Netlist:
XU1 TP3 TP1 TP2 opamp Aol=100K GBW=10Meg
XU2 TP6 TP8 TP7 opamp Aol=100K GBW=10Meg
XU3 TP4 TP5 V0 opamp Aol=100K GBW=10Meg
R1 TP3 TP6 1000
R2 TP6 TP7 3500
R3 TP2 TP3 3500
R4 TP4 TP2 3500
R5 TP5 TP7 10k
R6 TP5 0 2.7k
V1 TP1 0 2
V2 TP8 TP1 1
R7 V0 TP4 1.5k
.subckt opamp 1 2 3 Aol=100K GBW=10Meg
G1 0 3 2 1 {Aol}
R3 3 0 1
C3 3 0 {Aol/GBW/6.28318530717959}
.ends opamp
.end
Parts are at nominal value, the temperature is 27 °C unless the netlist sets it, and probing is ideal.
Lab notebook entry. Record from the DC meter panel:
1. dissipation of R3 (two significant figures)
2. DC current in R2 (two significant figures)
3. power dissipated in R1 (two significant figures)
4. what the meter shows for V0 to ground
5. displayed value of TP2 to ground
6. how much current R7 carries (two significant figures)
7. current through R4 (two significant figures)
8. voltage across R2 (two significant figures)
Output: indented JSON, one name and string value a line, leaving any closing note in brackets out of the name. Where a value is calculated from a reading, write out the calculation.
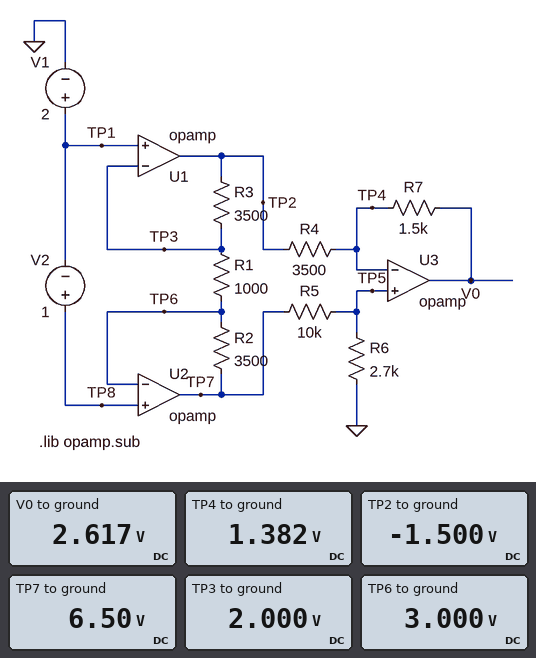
{
  "dissipation of R3": "(2 V - (-1.5 V))^2 / 3.5 kΩ = 3.5 mW",
  "DC current in R2": "(6.5 V - 3 V) / 3.5 kΩ = 1.0 mA",
  "power dissipated in R1": "(3 V - 2 V)^2 / 1 kΩ = 1.0 mW",
  "what the meter shows for V0 to ground": "2.617 V",
  "displayed value of TP2 to ground": "-1.500 V",
  "how much current R7 carries": "(2.617 V - 1.382 V) / 1.5 kΩ = 820 µA",
  "current through R4": "(1.382 V - (-1.5 V)) / 3.5 kΩ = 820 µA",
  "voltage across R2": "6.5 V - 3 V = 3.5 V"
}
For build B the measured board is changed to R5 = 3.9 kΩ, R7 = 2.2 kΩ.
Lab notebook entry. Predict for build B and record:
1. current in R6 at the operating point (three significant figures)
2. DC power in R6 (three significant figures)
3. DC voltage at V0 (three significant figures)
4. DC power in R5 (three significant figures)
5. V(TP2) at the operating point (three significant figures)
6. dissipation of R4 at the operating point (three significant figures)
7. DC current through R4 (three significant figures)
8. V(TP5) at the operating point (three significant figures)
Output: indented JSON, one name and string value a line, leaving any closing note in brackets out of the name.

{
  "current in R6 at the operating point": "985 µA",
  "DC power in R6": "2.62 mW",
  "DC voltage at V0": "5.27 V",
  "DC power in R5": "3.78 mW",
  "V(TP2) at the operating point": "-1.50 V",
  "dissipation of R4 at the operating point": "4.94 mW",
  "DC current through R4": "1.19 mA",
  "V(TP5) at the operating point": "2.66 V"
}
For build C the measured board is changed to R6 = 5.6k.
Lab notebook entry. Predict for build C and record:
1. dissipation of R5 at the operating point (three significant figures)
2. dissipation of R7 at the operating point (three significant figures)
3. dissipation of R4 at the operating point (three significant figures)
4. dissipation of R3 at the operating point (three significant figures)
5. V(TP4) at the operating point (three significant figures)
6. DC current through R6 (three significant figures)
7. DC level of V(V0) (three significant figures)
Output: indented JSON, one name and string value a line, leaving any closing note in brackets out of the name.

{
  "dissipation of R5 at the operating point": "1.74 mW",
  "dissipation of R7 at the operating point": "1.80 mW",
  "dissipation of R4 at the operating point": "4.20 mW",
  "dissipation of R3 at the operating point": "3.50 mW",
  "V(TP4) at the operating point": "2.33 V",
  "DC current through R6": "417 µA",
  "DC level of V(V0)": "3.98 V"
}
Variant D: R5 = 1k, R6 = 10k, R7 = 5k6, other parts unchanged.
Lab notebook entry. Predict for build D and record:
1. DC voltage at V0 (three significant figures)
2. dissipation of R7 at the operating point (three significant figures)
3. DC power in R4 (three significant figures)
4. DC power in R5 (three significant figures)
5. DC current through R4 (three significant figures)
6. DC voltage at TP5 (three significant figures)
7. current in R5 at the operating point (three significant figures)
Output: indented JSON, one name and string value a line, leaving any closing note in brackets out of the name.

{
  "DC voltage at V0": "17.8 V",
  "dissipation of R7 at the operating point": "25.1 mW",
  "DC power in R4": "15.7 mW",
  "DC power in R5": "349 µW",
  "DC current through R4": "2.12 mA",
  "DC voltage at TP5": "5.91 V",
  "current in R5 at the operating point": "591 µA"
}
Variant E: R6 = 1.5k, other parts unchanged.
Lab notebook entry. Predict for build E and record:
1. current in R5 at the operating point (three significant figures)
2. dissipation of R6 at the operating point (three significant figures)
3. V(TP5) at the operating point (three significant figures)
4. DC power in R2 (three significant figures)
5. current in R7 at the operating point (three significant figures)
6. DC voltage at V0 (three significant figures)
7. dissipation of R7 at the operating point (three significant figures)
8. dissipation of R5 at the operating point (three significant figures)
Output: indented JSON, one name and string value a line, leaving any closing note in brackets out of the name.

{
  "current in R5 at the operating point": "565 µA",
  "dissipation of R6 at the operating point": "479 µW",
  "V(TP5) at the operating point": "848 mV",
  "DC power in R2": "3.50 mW",
  "current in R7 at the operating point": "671 µA",
  "DC voltage at V0": "1.85 V",
  "dissipation of R7 at the operating point": "675 µW",
  "dissipation of R5 at the operating point": "3.19 mW"
}
